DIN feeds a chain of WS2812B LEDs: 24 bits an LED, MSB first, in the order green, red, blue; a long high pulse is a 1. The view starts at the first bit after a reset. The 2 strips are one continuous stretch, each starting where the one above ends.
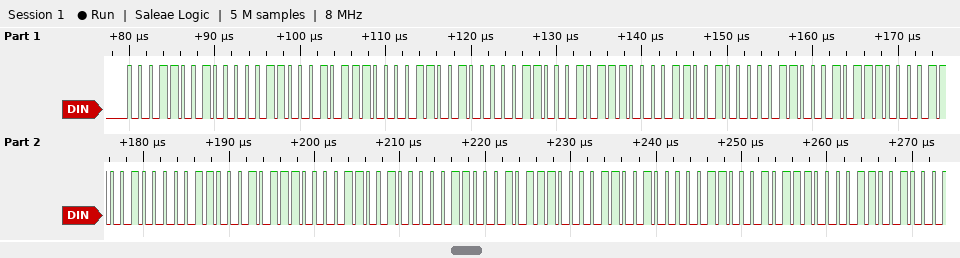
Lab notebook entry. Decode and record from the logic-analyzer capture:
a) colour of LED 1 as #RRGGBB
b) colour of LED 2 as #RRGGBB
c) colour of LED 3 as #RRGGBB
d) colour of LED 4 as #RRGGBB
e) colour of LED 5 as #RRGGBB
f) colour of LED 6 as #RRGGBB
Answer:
#06192E
#06192E
#06192E
#06192E
#06192E
#06192E
